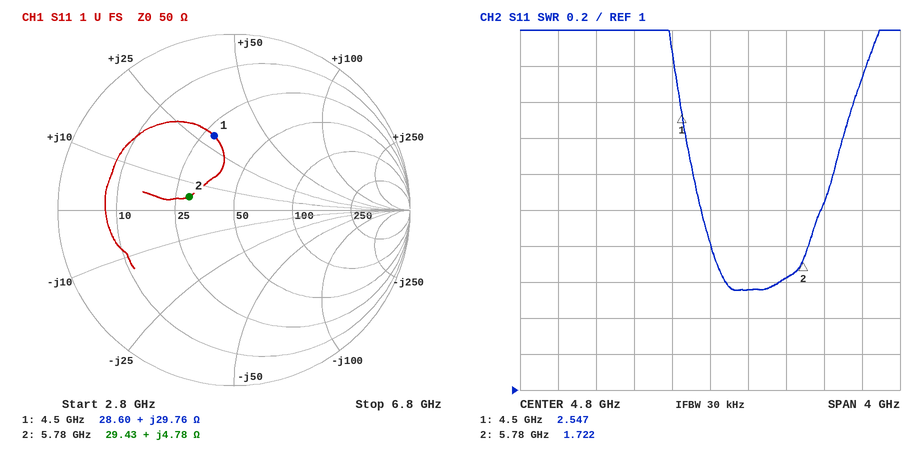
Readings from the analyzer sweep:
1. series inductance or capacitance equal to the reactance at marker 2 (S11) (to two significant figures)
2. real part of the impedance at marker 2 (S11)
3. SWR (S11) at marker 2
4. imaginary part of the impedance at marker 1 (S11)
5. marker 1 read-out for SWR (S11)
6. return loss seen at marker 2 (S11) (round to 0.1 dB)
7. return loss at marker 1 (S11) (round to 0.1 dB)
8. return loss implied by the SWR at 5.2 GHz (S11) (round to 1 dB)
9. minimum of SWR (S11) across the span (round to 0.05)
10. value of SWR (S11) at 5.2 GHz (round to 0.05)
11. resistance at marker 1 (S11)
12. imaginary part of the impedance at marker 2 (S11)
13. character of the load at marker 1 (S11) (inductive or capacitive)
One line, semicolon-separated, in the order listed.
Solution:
130 pH; 29.43 Ω; 1.722; +29.76 Ω; 2.547; 11.5 dB; 7.2 dB; 13 dB; 1.55; 1.55; 28.60 Ω; +4.78 Ω; inductive
